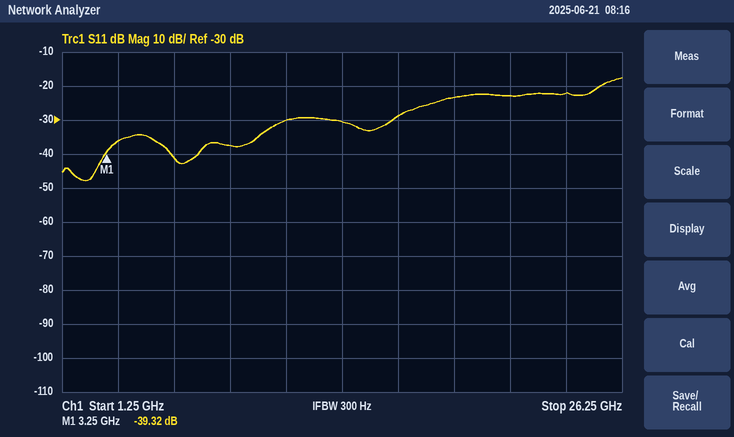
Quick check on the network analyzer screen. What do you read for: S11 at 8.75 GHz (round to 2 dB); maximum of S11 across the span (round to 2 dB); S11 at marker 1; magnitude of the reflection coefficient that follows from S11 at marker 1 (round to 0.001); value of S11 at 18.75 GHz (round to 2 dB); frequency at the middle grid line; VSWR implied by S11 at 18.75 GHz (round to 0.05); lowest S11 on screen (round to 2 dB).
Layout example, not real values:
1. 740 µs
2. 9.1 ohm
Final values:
1. -38 dB
2. -18 dB
3. -39.32 dB
4. 0.011
5. -24 dB
6. 13.75 GHz
7. 1.15
8. -48 dB
